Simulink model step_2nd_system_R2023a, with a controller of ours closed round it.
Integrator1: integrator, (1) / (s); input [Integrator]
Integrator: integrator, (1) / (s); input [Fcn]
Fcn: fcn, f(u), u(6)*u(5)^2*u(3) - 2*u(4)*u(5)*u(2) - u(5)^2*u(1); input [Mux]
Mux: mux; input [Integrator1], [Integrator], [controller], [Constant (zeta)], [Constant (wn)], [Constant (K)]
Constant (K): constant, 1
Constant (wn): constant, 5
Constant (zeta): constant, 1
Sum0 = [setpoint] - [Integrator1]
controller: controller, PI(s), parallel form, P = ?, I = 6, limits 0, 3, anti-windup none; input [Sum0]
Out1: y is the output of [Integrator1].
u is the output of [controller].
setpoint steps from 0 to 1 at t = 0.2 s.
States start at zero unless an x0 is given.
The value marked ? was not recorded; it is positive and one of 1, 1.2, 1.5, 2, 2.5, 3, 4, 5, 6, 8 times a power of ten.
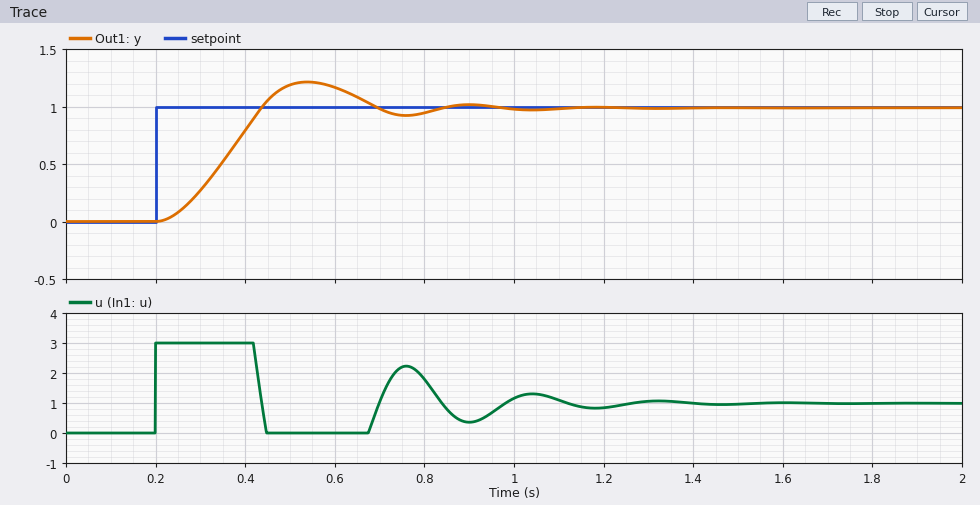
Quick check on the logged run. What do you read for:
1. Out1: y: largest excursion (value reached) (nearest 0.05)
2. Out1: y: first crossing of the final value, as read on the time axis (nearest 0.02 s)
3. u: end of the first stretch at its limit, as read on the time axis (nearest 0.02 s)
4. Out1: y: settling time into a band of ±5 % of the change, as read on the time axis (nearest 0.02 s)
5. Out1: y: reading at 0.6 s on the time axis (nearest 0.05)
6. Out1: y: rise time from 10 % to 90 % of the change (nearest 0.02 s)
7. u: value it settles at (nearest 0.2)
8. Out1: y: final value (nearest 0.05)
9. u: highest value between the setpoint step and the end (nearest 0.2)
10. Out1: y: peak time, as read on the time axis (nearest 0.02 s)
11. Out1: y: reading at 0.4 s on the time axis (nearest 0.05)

1.20
0.44 s
0.42 s
0.80 s
1.15
0.16 s
1.0
1.00
3.0
0.54 s
0.80
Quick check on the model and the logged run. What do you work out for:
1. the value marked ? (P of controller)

20
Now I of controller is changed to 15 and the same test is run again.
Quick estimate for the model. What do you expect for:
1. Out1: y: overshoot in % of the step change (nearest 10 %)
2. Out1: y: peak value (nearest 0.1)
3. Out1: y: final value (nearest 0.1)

30 %
1.3
1.0
